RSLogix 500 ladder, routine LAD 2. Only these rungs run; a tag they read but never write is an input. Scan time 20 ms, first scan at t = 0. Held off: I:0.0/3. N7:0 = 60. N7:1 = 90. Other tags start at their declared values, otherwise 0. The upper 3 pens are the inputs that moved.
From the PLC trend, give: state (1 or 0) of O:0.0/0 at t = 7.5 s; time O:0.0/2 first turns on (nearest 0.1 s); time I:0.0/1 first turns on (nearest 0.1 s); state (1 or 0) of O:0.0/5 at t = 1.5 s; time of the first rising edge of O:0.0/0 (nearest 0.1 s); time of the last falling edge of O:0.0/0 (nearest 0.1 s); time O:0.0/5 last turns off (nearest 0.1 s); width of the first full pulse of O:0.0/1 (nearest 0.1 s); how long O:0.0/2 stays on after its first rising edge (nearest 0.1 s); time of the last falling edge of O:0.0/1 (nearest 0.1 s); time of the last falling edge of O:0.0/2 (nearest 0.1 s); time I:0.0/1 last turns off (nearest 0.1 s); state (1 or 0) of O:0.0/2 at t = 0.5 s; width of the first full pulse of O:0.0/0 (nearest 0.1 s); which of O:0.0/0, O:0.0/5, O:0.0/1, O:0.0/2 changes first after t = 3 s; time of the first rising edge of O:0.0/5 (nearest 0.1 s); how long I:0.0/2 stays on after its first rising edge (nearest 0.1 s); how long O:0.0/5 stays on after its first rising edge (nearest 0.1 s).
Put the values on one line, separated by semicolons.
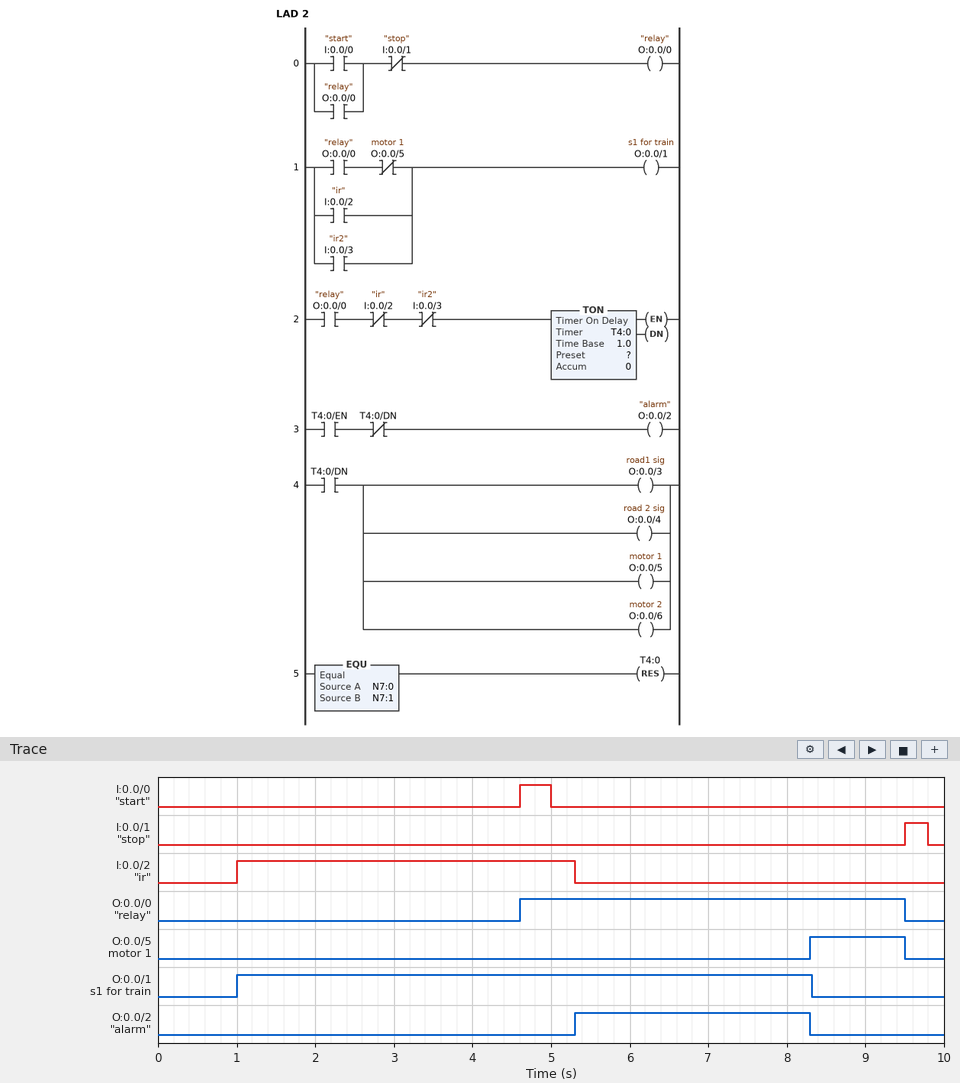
1; 5.3 s; 9.5 s; 0; 4.6 s; 9.5 s; 9.5 s; 7.3 s; 3.0 s; 8.3 s; 8.3 s; 9.8 s; 0; 4.9 s; O:0.0/0; 8.3 s; 4.3 s; 1.2 s
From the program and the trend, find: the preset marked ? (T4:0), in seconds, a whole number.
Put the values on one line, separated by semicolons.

3 s
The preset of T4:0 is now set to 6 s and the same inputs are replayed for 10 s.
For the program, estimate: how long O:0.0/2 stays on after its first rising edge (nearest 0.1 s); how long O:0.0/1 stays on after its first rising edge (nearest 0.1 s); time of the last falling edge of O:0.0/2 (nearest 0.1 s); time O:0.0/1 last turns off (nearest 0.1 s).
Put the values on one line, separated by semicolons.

4.2 s; 8.5 s; 9.5 s; 9.5 s
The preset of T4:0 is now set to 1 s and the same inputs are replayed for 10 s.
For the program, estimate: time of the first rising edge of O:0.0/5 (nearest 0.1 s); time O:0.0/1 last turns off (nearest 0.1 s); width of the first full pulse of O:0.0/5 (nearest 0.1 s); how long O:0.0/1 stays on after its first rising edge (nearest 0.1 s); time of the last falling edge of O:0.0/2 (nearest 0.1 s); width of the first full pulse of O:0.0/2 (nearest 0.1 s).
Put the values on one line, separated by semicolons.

6.3 s; 6.3 s; 3.2 s; 5.3 s; 6.3 s; 1.0 s
